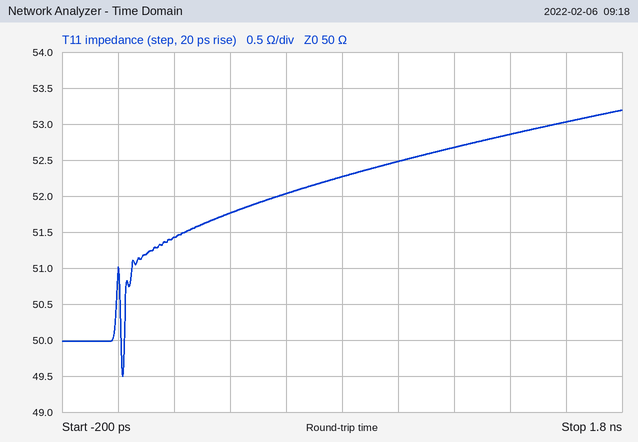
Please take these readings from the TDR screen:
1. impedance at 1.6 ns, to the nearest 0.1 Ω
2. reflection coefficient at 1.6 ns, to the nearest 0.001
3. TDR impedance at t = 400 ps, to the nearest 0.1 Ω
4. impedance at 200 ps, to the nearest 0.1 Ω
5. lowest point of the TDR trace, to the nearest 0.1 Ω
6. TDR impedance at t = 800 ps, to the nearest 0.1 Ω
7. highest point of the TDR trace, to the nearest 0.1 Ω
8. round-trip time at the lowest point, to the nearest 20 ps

53.0 Ω
+0.029
51.8 Ω
51.4 Ω
49.5 Ω
52.3 Ω
53.2 Ω
20 ps
